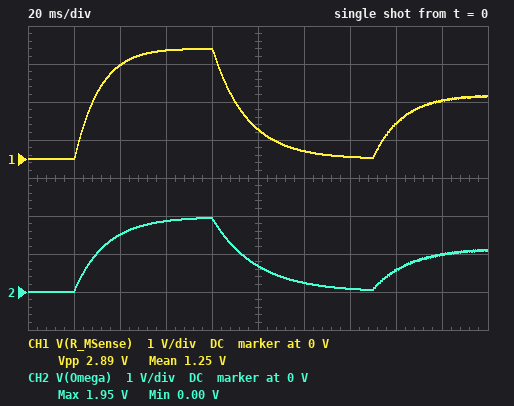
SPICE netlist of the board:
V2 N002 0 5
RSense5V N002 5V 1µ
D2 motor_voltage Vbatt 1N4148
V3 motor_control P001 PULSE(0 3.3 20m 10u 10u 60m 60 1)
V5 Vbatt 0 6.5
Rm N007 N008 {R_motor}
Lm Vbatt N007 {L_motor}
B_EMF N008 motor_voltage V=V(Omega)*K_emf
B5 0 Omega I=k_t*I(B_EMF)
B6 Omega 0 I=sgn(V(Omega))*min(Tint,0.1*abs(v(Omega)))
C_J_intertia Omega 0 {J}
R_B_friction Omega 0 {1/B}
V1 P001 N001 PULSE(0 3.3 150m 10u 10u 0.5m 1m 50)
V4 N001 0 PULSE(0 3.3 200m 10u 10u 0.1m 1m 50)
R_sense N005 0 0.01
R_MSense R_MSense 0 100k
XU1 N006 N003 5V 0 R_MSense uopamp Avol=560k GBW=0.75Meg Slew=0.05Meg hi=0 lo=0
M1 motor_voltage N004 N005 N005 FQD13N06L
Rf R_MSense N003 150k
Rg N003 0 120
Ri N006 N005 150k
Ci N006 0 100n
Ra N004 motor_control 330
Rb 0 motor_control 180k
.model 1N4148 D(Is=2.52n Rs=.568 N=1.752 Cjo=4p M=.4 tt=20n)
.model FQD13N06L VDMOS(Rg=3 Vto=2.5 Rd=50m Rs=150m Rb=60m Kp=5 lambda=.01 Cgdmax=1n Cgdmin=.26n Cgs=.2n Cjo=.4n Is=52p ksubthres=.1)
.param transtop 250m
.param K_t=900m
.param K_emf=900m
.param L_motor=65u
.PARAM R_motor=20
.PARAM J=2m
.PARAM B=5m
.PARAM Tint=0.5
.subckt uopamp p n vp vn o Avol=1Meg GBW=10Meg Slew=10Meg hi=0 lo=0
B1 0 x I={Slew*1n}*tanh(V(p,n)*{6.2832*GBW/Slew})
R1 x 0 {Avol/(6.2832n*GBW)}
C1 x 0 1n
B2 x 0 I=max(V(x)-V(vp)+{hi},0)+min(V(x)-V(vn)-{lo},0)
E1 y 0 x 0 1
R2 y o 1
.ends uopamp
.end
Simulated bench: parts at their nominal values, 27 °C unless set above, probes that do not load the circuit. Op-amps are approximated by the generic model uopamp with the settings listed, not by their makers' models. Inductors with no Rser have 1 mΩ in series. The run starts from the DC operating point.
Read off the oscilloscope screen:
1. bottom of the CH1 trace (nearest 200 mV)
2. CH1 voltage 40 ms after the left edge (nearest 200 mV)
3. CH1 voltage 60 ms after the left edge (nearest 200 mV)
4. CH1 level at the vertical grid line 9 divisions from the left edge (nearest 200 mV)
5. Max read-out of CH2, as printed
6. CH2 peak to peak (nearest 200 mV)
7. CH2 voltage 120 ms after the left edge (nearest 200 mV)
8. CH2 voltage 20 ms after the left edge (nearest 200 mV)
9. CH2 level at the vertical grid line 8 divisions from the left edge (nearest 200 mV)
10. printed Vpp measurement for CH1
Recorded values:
0 V
2.4 V
2.8 V
1.6 V
1.95 V
2.0 V
200 mV
0 V
600 mV
2.89 V
